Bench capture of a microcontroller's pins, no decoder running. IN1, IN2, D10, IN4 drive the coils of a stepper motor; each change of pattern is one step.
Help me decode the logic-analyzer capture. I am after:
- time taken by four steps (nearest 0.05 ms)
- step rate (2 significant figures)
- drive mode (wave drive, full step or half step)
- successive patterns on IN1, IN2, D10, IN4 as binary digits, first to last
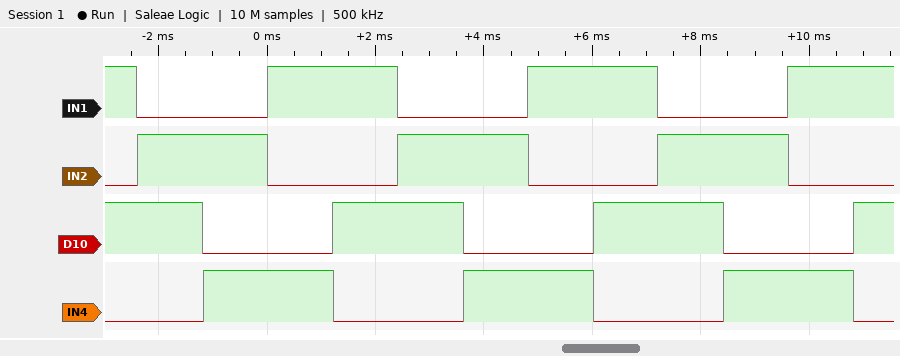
4.80 ms
830 steps/s
full step
1010 0110 0101 1001 1010 0110 0101 1001 1010 0110 0101 1001 1010
